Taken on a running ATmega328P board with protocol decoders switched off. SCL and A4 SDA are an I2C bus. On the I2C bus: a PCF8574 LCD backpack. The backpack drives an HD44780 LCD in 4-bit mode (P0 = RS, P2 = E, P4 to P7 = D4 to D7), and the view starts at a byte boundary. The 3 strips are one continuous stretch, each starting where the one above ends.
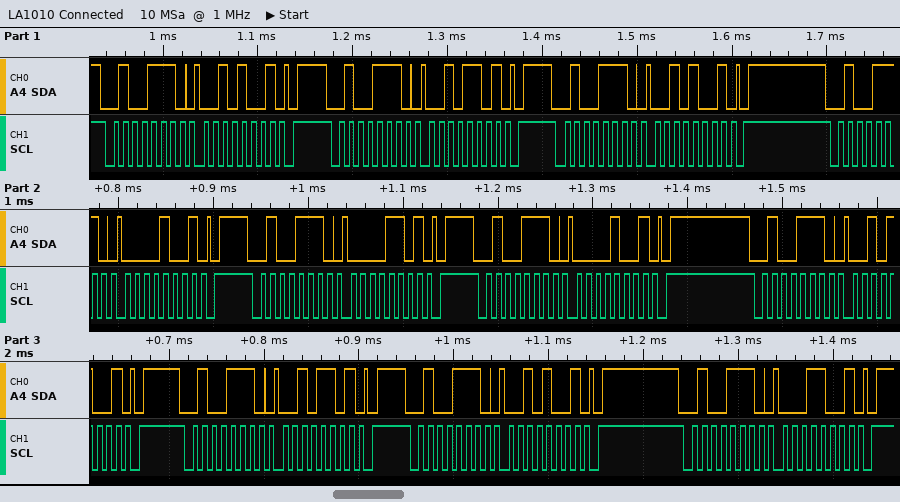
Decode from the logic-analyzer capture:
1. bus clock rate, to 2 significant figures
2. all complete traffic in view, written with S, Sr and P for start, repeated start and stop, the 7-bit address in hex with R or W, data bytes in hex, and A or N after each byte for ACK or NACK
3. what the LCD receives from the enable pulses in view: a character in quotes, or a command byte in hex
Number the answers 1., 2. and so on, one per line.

1. 100 kHz
2. S 27W A 29 A P S 27W A 2D A P S 27W A 29 A P S 27W A 09 A P S 27W A 0D A P S 27W A 09 A P S 27W A 29 A P S 27W A 2D A P S 27W A 29 A P S 27W A 19 A P
3. ' '
